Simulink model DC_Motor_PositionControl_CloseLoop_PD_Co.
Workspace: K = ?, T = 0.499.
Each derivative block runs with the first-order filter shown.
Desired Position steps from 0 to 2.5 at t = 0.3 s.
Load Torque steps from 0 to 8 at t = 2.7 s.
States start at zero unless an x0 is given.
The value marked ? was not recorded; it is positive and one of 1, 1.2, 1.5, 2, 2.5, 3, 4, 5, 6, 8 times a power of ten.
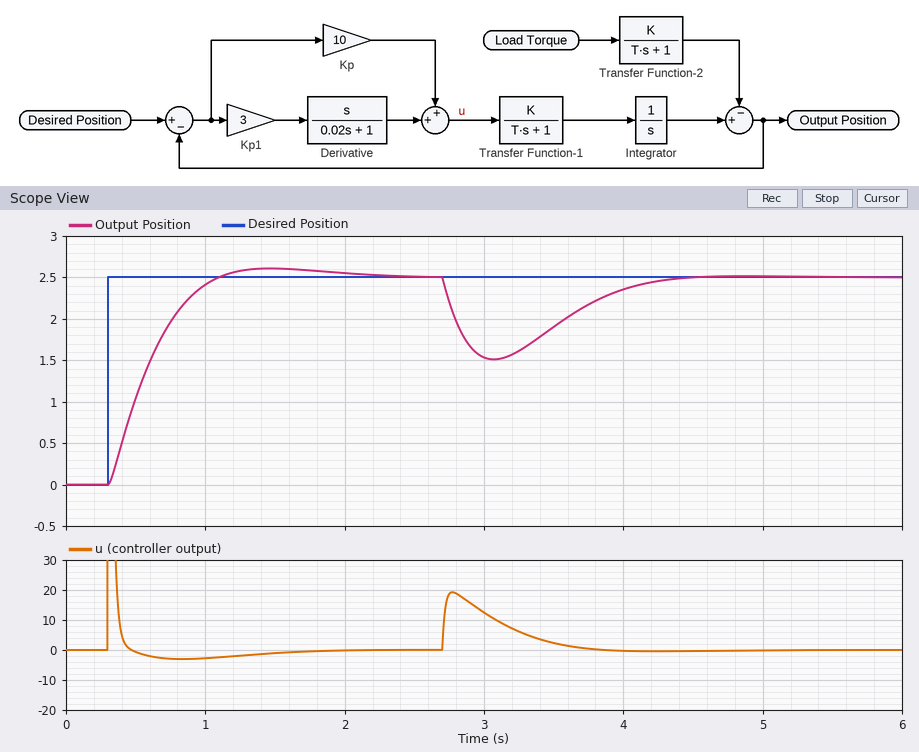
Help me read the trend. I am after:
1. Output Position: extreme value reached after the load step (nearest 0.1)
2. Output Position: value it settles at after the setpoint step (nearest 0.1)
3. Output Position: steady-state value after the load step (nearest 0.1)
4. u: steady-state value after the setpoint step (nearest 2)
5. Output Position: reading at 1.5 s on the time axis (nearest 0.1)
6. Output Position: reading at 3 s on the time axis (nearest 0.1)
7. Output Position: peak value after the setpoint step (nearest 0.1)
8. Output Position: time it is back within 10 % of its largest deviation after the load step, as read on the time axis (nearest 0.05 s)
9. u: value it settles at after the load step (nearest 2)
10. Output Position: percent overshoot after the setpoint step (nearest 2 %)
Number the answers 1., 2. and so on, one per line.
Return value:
1. 1.5
2. 2.5
3. 2.5
4. 0
5. 2.6
6. 1.5
7. 2.6
8. 4.10 s
9. 0
10. 4 %
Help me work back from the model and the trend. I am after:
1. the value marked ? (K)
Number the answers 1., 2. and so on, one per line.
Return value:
1. 0.4
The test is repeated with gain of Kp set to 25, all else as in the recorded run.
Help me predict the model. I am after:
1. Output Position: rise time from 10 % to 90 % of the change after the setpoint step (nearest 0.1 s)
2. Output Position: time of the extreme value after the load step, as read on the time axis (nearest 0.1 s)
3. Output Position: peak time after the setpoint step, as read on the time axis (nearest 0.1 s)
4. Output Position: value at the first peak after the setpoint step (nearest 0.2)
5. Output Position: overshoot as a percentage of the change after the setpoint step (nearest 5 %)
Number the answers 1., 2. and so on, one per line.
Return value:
1. 0.3 s
2. 3.0 s
3. 0.9 s
4. 3.0
5. 20 %
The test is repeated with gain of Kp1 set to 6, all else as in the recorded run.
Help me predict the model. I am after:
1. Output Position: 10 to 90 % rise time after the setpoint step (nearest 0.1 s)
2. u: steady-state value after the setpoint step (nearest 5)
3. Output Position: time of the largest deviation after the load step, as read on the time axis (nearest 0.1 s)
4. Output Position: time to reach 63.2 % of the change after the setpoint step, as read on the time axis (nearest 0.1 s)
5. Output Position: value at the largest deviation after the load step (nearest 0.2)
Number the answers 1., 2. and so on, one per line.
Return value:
1. 0.5 s
2. 0
3. 3.0 s
4. 0.5 s
5. 1.8
